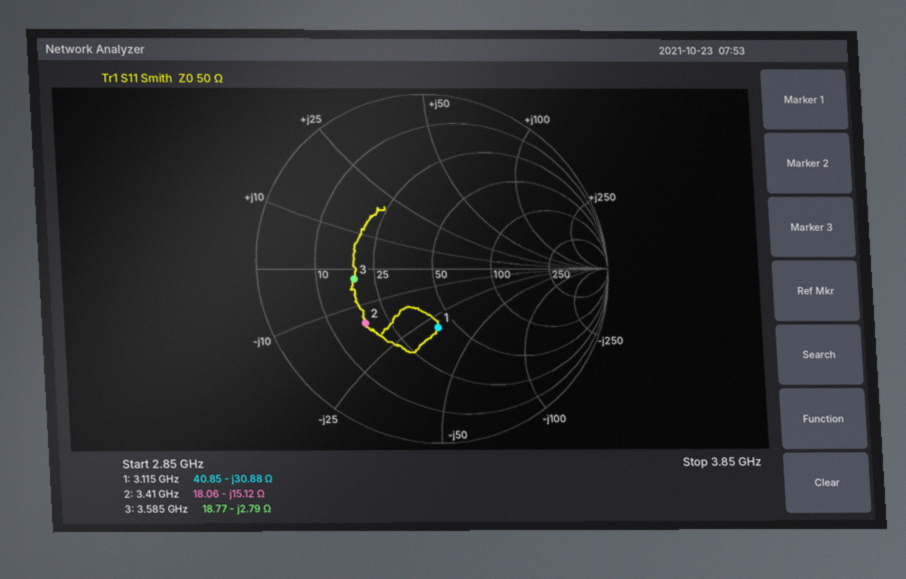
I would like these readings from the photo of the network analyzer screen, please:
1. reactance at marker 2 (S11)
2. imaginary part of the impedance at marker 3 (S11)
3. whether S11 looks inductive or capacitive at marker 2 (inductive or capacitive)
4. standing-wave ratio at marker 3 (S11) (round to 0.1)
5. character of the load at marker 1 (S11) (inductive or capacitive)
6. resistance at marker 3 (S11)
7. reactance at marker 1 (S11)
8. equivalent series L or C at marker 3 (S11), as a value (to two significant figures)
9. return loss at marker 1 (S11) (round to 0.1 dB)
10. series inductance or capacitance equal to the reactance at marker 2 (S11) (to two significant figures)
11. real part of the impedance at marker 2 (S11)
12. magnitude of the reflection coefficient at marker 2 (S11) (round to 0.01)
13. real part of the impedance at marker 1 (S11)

-15.12 Ω
-2.79 Ω
capacitive
2.7
capacitive
18.77 Ω
-30.88 Ω
16 pF
9.5 dB
3.1 pF
18.06 Ω
0.51
40.85 Ω
